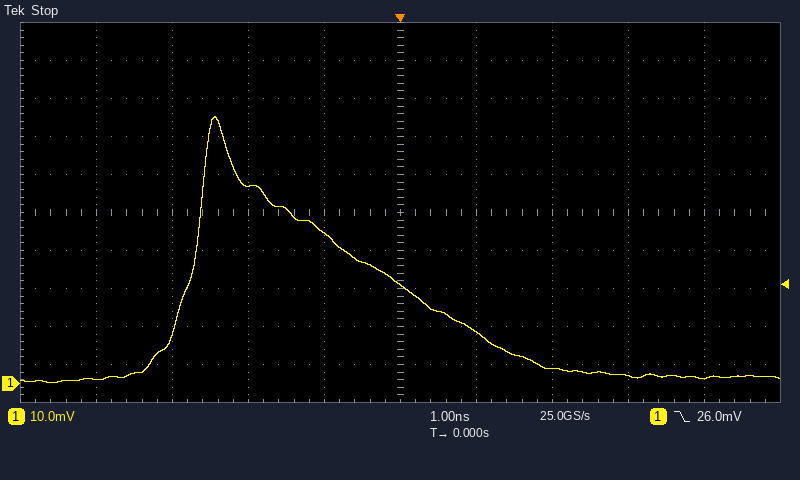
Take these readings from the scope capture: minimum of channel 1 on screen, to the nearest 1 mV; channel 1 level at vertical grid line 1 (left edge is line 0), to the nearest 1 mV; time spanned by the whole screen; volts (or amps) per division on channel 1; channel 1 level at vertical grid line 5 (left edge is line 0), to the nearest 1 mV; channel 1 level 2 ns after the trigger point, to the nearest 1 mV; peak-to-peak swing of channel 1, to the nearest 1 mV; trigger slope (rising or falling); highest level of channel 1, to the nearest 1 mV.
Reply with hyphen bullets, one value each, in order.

- 0 mV
- 1 mV
- 10 ns
- 10 mV
- 26 mV
- 4 mV
- 70 mV
- falling
- 70 mV
